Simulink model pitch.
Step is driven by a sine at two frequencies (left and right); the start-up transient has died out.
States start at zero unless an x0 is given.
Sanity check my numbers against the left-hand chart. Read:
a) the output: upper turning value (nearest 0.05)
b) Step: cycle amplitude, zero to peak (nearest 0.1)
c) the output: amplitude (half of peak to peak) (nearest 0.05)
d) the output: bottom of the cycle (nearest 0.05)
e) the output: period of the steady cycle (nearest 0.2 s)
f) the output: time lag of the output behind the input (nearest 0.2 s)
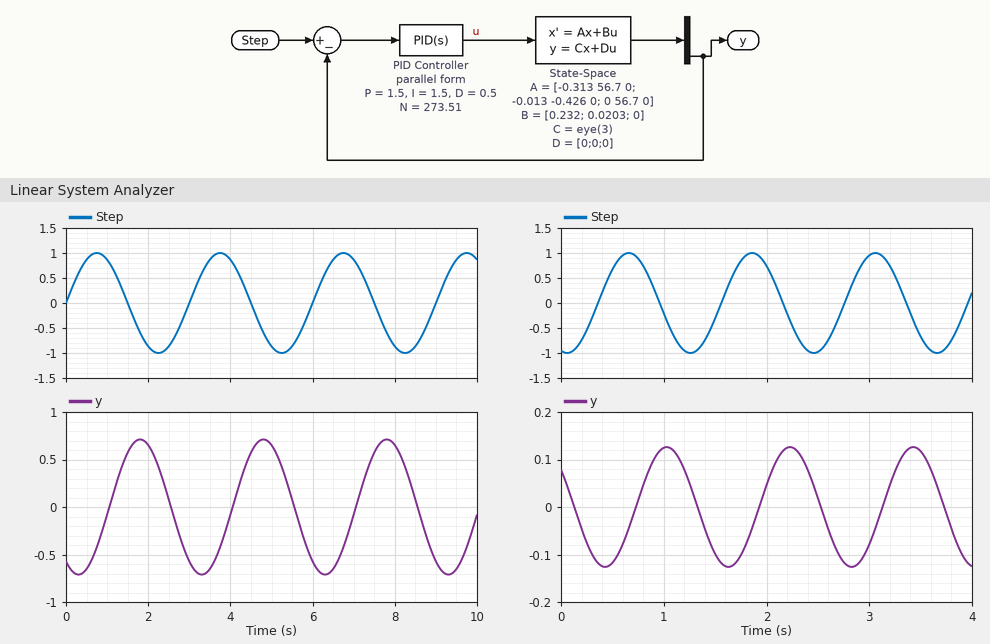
0.70
1.0
0.70
-0.70
3.0 s
1.0 s
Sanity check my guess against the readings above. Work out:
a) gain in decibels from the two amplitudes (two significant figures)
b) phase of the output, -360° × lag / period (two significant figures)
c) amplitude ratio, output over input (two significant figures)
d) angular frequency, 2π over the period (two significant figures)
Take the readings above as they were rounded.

-3.1 dB
-120°
0.70
2.1 rad/s
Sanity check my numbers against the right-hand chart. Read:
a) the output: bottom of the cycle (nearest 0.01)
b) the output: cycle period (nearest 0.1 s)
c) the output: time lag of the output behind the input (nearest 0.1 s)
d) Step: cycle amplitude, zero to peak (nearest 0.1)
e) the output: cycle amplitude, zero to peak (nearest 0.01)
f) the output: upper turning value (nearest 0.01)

-0.13
1.2 s
0.4 s
1.0
0.13
0.13
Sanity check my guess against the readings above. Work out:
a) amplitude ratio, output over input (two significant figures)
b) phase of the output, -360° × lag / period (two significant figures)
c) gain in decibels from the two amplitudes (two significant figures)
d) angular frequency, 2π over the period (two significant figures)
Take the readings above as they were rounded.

0.13
-120°
-18 dB
5.2 rad/s
